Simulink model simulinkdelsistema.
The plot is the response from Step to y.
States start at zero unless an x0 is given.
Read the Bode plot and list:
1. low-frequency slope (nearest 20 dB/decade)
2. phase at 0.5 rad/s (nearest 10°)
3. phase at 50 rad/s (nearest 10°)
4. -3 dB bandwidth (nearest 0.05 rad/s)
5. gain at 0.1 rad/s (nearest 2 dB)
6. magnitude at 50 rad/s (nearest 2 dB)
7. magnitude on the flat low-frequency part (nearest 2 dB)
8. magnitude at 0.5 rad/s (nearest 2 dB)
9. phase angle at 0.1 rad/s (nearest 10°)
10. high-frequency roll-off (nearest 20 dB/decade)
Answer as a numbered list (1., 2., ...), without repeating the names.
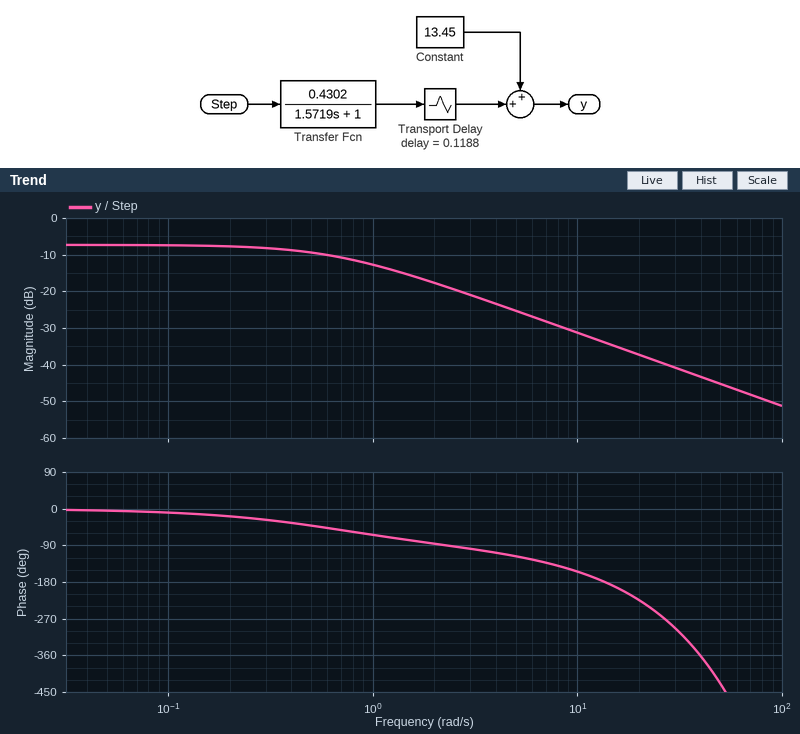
1. 0 dB/decade
2. -40°
3. -430°
4. 0.65 rad/s
5. -8 dB
6. -46 dB
7. -8 dB
8. -10 dB
9. -10°
10. -20 dB/decade
